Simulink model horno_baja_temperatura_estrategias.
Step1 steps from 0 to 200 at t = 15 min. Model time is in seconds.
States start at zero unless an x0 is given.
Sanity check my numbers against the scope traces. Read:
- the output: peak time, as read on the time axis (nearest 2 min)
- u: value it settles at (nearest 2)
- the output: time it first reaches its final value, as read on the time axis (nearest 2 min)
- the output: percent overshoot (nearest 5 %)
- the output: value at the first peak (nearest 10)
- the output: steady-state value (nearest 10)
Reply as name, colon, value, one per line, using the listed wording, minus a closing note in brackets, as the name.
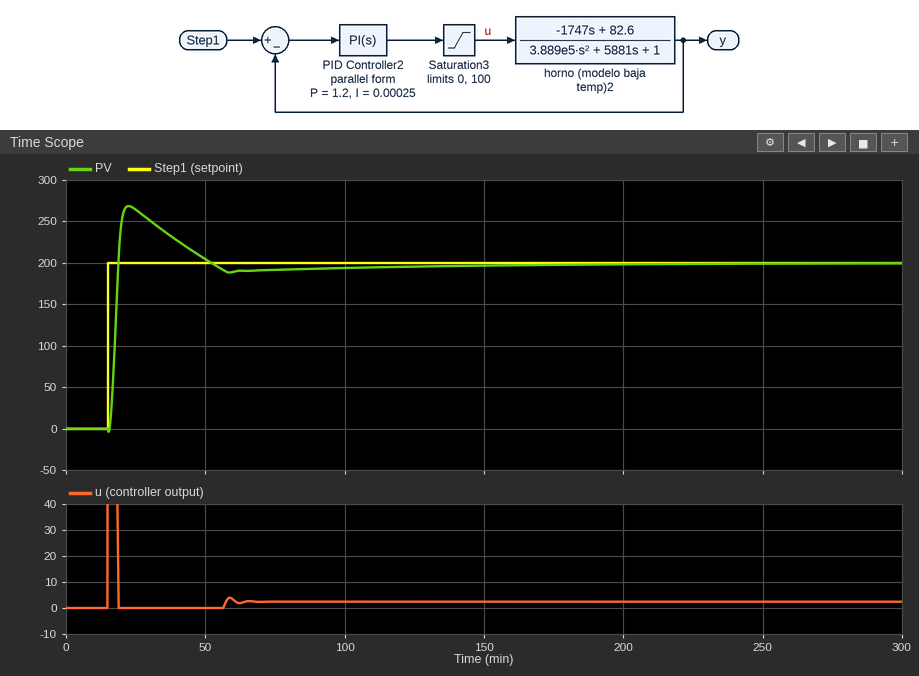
the output: peak time, as read on the time axis: 22 min
u: value it settles at: 2
the output: time it first reaches its final value, as read on the time axis: 18 min
the output: percent overshoot: 35 %
the output: value at the first peak: 270
the output: steady-state value: 200
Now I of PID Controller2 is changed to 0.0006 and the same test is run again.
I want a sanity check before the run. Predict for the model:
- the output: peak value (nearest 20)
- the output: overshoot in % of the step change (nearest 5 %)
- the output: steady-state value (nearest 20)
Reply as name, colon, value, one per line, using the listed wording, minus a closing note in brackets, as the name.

the output: peak value: 280
the output: overshoot in % of the step change: 40 %
the output: steady-state value: 200
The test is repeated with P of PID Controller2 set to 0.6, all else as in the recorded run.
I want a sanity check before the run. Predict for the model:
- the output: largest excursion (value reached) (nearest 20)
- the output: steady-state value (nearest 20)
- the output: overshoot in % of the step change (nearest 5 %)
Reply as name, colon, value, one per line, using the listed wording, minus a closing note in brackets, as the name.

the output: largest excursion (value reached): 240
the output: steady-state value: 200
the output: overshoot in % of the step change: 20 %
